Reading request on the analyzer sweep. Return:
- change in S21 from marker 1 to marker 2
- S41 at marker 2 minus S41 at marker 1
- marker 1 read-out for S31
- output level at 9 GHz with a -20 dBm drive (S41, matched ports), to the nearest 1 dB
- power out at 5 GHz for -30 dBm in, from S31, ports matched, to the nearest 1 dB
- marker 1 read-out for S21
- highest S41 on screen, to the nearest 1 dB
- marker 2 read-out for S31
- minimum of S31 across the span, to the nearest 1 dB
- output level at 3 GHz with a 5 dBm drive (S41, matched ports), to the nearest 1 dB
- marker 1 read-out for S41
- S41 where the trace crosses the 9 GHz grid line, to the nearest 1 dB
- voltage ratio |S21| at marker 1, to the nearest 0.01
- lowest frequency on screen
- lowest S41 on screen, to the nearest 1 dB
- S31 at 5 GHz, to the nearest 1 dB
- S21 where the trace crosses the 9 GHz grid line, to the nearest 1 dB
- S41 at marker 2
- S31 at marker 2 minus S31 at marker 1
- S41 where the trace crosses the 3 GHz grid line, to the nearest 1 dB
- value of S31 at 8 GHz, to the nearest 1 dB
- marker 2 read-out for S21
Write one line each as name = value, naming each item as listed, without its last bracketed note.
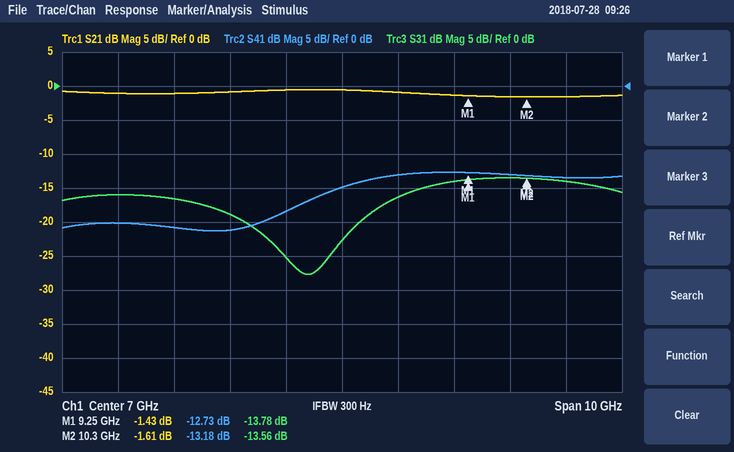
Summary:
change in S21 from marker 1 to marker 2 = -0.18 dB
S41 at marker 2 minus S41 at marker 1 = -0.45 dB
marker 1 read-out for S31 = -13.78 dB
output level at 9 GHz with a -20 dBm drive (S41, matched ports), to the nearest 1 dB = -33 dBm
power out at 5 GHz for -30 dBm in, from S31, ports matched, to the nearest 1 dB = -49 dBm
marker 1 read-out for S21 = -1.43 dB
highest S41 on screen, to the nearest 1 dB = -13 dB
marker 2 read-out for S31 = -13.56 dB
minimum of S31 across the span, to the nearest 1 dB = -28 dB
output level at 3 GHz with a 5 dBm drive (S41, matched ports), to the nearest 1 dB = -15 dBm
marker 1 read-out for S41 = -12.73 dB
S41 where the trace crosses the 9 GHz grid line, to the nearest 1 dB = -13 dB
voltage ratio |S21| at marker 1, to the nearest 0.01 = 0.85
lowest frequency on screen = 2 GHz
lowest S41 on screen, to the nearest 1 dB = -21 dB
S31 at 5 GHz, to the nearest 1 dB = -19 dB
S21 where the trace crosses the 9 GHz grid line, to the nearest 1 dB = -1 dB
S41 at marker 2 = -13.18 dB
S31 at marker 2 minus S31 at marker 1 = 0.22 dB
S41 where the trace crosses the 3 GHz grid line, to the nearest 1 dB = -20 dB
value of S31 at 8 GHz, to the nearest 1 dB = -16 dB
marker 2 read-out for S21 = -1.61 dB
